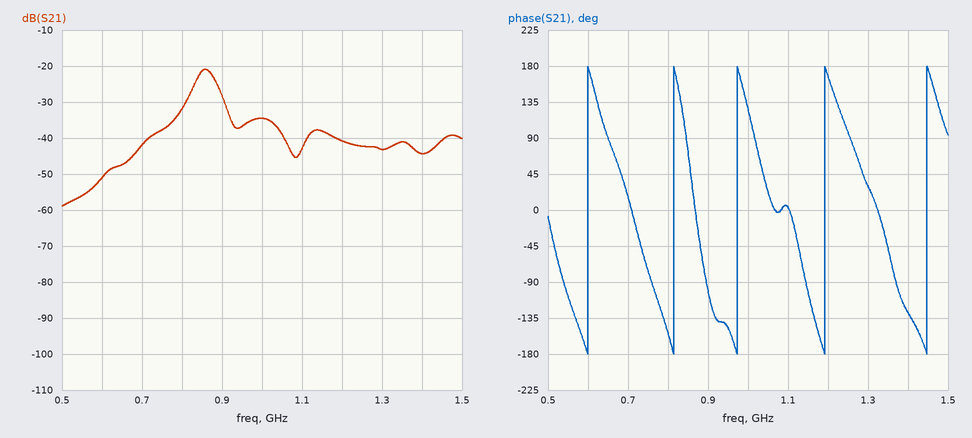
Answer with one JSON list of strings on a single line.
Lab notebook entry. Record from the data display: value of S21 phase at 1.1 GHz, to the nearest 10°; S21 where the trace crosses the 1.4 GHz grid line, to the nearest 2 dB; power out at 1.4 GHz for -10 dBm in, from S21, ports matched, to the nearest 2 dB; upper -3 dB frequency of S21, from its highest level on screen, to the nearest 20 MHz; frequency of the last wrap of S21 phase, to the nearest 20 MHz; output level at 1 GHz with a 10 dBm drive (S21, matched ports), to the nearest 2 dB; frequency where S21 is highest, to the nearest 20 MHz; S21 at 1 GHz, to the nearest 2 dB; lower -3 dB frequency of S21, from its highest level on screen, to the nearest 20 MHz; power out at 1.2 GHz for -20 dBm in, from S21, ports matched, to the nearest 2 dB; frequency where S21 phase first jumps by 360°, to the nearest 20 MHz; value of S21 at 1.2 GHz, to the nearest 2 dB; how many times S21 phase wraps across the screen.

["0°", "-44 dB", "-54 dBm", "880 MHz", "1.44 GHz", "-24 dBm", "860 MHz", "-34 dB", "840 MHz", "-60 dBm", "600 MHz", "-40 dB", "5"]
